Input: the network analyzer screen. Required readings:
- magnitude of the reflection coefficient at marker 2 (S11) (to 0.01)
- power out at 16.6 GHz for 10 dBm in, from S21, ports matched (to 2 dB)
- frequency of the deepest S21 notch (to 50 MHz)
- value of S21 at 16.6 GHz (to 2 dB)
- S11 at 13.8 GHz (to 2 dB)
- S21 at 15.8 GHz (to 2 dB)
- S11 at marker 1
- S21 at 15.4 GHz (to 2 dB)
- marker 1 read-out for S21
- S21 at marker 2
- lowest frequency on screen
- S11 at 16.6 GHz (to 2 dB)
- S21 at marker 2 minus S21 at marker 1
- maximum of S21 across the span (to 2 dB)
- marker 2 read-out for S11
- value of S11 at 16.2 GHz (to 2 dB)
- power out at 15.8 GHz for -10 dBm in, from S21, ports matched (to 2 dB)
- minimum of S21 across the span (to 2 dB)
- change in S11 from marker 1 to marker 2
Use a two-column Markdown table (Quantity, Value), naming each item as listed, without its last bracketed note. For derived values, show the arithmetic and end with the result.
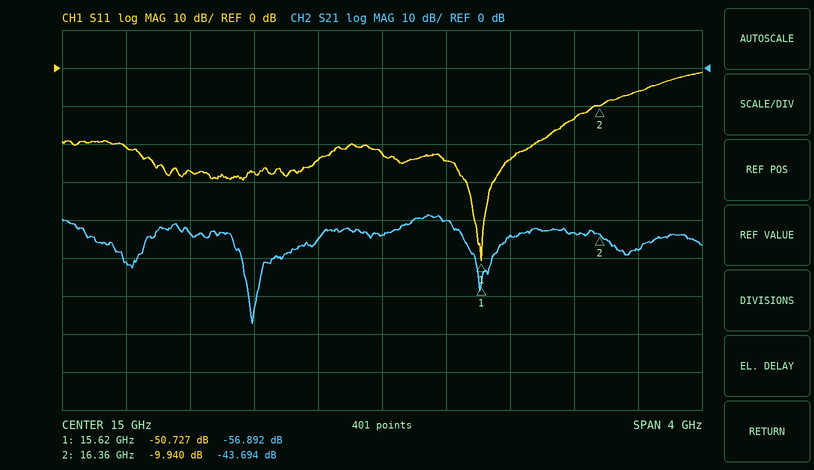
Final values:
| Quantity | Value |
|---|---|
| magnitude of the reflection coefficient at marker 2 (S11) | 10^(-9.94/20) ≈ 0.32 |
| power out at 16.6 GHz for 10 dBm in, from S21, ports matched | 10 dBm + (-48 dB) = -38 dBm |
| frequency of the deepest S21 notch | 14.20 GHz |
| value of S21 at 16.6 GHz | -48 dB |
| S11 at 13.8 GHz | -28 dB |
| S21 at 15.8 GHz | -44 dB |
| S11 at marker 1 | -50.727 dB |
| S21 at 15.4 GHz | -40 dB |
| marker 1 read-out for S21 | -56.892 dB |
| S21 at marker 2 | -43.694 dB |
| lowest frequency on screen | 13 GHz |
| S11 at 16.6 GHz | -6 dB |
| S21 at marker 2 minus S21 at marker 1 | -43.694 − (-56.892) = 13.198 dB |
| maximum of S21 across the span | -38 dB |
| marker 2 read-out for S11 | -9.940 dB |
| value of S11 at 16.2 GHz | -14 dB |
| power out at 15.8 GHz for -10 dBm in, from S21, ports matched | -10 dBm + (-44 dB) = -54 dBm |
| minimum of S21 across the span | -68 dB |
| change in S11 from marker 1 to marker 2 | -9.94 − (-50.727) = 40.787 dB |
